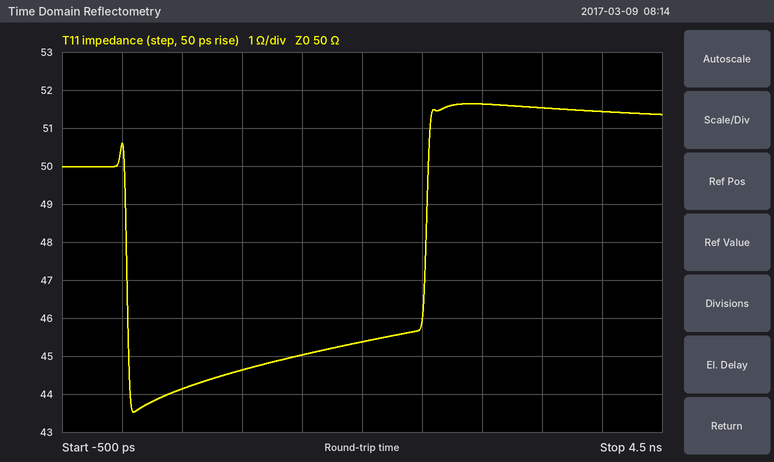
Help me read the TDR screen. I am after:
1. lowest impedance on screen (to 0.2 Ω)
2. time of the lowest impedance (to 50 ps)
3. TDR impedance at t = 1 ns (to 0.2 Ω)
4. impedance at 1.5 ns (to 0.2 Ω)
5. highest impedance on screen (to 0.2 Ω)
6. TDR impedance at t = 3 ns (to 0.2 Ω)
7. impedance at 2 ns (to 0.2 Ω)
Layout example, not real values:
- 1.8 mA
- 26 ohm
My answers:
- 43.6 Ω
- 100 ps
- 44.6 Ω
- 45.0 Ω
- 51.6 Ω
- 51.6 Ω
- 45.4 Ω
